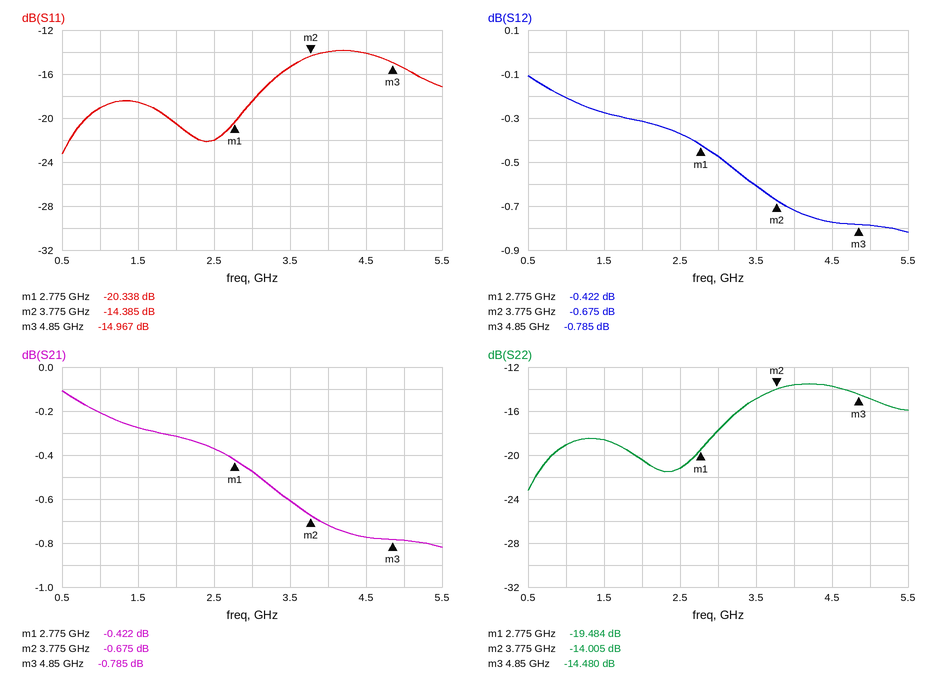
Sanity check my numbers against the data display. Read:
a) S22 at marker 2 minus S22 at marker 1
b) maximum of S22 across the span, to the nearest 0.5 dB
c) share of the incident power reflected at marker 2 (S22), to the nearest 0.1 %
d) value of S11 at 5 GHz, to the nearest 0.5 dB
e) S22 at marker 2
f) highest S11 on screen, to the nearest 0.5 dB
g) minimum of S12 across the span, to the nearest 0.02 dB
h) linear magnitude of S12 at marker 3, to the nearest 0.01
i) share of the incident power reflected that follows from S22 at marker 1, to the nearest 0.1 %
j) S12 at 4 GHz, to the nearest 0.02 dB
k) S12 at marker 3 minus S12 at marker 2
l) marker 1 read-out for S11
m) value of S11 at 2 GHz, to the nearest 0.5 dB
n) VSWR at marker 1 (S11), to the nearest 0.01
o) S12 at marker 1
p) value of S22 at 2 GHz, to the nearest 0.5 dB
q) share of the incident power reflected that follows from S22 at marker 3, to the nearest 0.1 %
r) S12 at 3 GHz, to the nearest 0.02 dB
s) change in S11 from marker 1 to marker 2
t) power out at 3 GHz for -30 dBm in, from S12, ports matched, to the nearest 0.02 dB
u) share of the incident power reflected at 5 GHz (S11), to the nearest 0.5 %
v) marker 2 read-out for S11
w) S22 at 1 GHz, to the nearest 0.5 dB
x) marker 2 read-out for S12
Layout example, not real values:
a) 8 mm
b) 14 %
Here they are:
a) 5.479 dB
b) -13.5 dB
c) 4.0 %
d) -15.5 dB
e) -14.005 dB
f) -14.0 dB
g) -0.82 dB
h) 0.91
i) 1.1 %
j) -0.72 dB
k) -0.110 dB
l) -20.338 dB
m) -20.5 dB
n) 1.21
o) -0.422 dB
p) -20.5 dB
q) 3.6 %
r) -0.48 dB
s) 5.953 dB
t) -30.48 dBm
u) 3.0 %
v) -14.385 dB
w) -19.0 dB
x) -0.675 dB
